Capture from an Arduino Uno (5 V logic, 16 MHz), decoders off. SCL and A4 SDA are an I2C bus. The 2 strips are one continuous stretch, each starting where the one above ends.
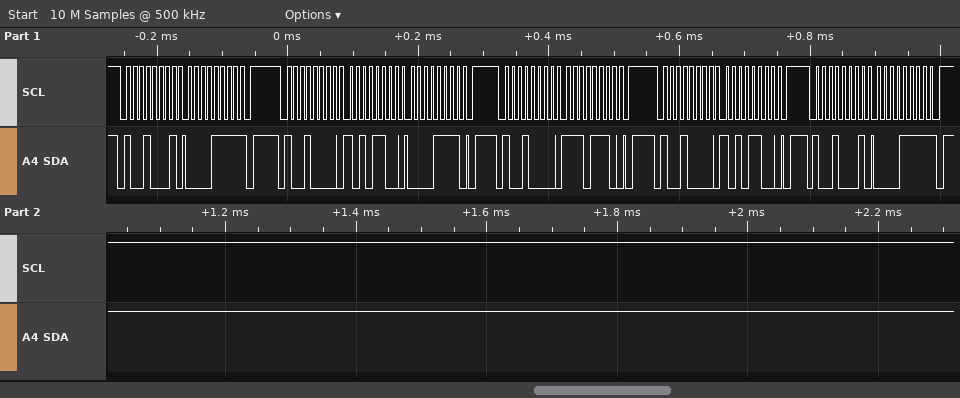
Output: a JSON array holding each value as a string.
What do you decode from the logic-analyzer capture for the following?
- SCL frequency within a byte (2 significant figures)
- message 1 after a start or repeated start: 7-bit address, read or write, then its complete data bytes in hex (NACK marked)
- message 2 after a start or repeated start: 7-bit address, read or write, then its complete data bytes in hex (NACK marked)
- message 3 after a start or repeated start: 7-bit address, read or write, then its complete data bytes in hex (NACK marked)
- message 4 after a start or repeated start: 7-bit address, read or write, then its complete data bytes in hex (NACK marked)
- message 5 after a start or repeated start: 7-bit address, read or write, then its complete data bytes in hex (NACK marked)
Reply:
["100 kHz", "0x48 read: 0F NACK", "0x48 write: AC 0F", "0x48 write: EE", "0x48 write: AC", "0x48 read: 0F NACK"]
